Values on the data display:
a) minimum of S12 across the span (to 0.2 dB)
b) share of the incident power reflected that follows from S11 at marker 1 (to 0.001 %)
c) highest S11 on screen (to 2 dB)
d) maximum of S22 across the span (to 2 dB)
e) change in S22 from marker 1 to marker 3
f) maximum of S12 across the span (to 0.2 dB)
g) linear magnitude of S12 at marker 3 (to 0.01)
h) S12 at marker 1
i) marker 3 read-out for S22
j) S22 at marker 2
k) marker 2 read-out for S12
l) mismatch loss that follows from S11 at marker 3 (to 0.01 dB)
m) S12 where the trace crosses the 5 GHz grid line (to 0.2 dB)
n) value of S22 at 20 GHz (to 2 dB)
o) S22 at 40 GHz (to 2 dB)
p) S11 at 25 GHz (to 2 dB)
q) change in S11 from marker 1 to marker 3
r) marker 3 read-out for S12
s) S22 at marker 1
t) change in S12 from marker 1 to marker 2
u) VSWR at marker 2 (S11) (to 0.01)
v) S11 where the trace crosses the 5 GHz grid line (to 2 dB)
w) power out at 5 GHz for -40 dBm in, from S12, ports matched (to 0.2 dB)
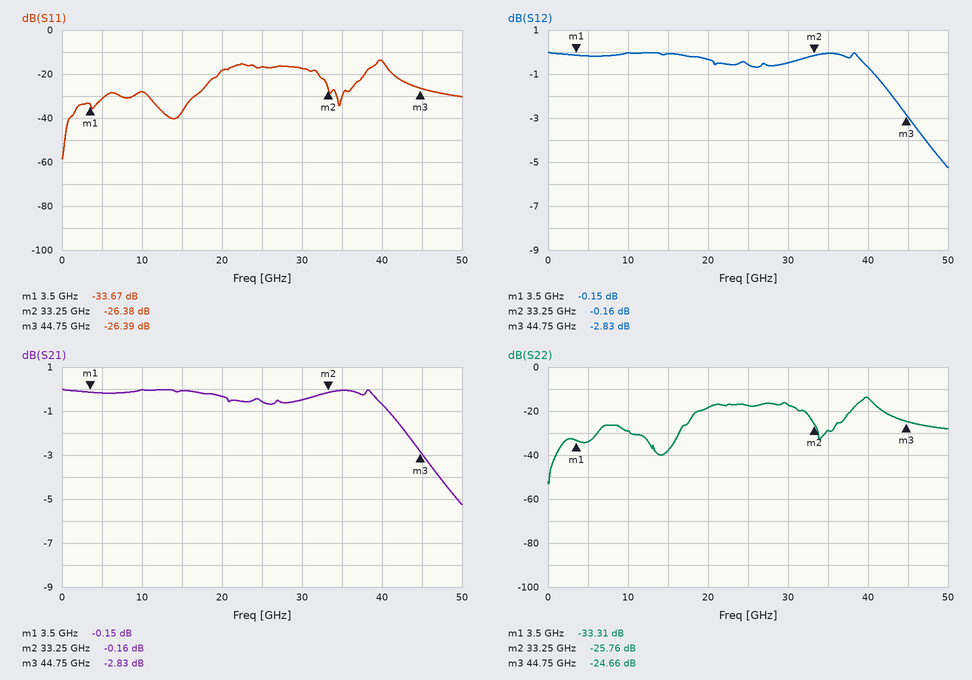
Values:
-5.2 dB
0.043 %
-14 dB
-14 dB
8.65 dB
0.0 dB
0.72
-0.15 dB
-24.66 dB
-25.76 dB
-0.16 dB
0.01 dB
-0.2 dB
-18 dB
-14 dB
-16 dB
7.28 dB
-2.83 dB
-33.31 dB
-0.01 dB
1.10
-32 dB
-40.2 dBm
